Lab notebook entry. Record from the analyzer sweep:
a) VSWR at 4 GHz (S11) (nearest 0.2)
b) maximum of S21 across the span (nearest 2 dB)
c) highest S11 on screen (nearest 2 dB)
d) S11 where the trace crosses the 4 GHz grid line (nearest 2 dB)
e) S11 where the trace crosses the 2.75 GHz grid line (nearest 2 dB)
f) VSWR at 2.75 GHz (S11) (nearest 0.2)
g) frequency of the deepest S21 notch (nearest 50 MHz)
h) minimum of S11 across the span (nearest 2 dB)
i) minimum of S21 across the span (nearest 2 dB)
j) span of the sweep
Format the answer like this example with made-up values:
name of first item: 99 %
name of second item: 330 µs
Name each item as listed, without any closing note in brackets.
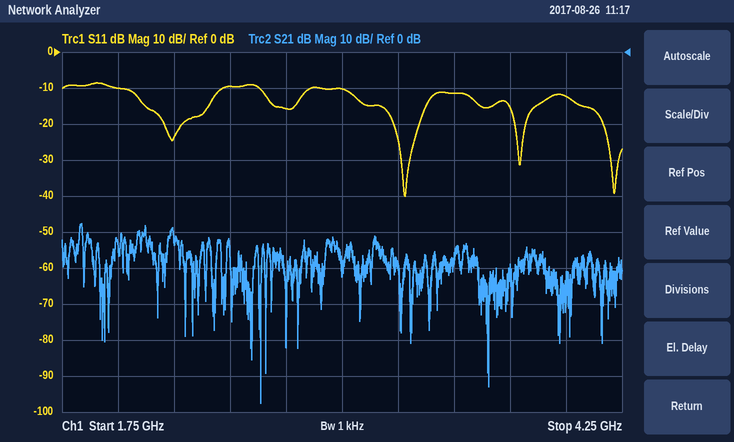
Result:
VSWR at 4 GHz (S11): 1.6
maximum of S21 across the span: -48 dB
highest S11 on screen: -8 dB
S11 where the trace crosses the 4 GHz grid line: -12 dB
S11 where the trace crosses the 2.75 GHz grid line: -16 dB
VSWR at 2.75 GHz (S11): 1.4
frequency of the deepest S21 notch: 2.65 GHz
minimum of S11 across the span: -40 dB
minimum of S21 across the span: -98 dB
span of the sweep: 2.5 GHz
